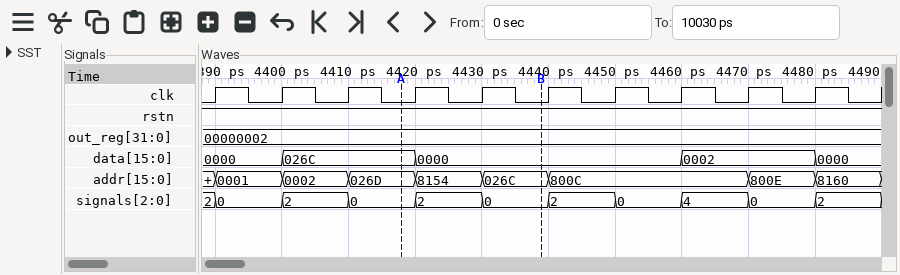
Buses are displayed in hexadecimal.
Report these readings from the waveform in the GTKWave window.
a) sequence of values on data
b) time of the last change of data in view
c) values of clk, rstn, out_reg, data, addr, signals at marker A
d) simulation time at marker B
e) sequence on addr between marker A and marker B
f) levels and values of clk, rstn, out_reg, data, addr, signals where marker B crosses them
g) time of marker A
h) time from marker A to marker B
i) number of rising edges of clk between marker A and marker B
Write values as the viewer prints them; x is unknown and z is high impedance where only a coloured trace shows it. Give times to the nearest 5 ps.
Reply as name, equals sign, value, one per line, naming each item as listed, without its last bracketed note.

sequence of values on data = 0000, 026C, 0000, 0002, 0000
time of the last change of data in view = 4480 ps
values of clk, rstn, out_reg, data, addr, signals at marker A = clk=0, rstn=1, out_reg=00000002, data=026C, addr=026D, signals=0
simulation time at marker B = 4440 ps
sequence on addr between marker A and marker B = 026D, 8154, 026C
levels and values of clk, rstn, out_reg, data, addr, signals where marker B crosses them = clk=0, rstn=1, out_reg=00000002, data=0000, addr=026C, signals=0
time of marker A = 4420 ps
time from marker A to marker B = 20 ps
number of rising edges of clk between marker A and marker B = 2
